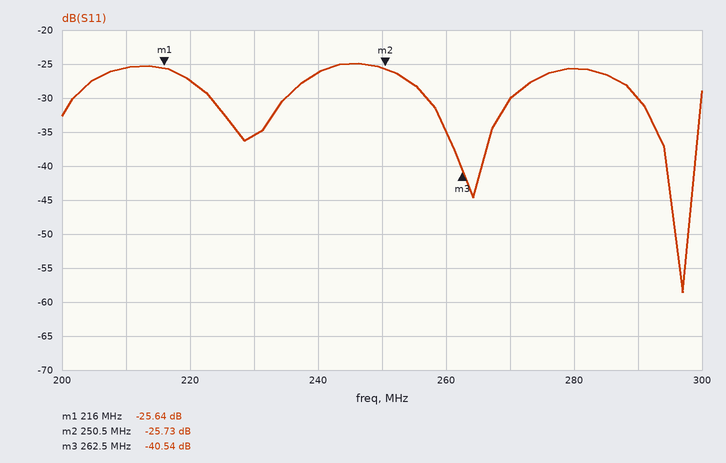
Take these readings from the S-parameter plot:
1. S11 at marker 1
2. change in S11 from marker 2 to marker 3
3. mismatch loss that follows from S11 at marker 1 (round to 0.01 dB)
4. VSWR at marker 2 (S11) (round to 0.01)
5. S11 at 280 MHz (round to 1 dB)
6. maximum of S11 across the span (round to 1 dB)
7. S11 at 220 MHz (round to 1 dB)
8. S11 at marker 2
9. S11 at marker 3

-25.64 dB
-14.81 dB
0.01 dB
1.11
-26 dB
-25 dB
-27 dB
-25.73 dB
-40.54 dB
